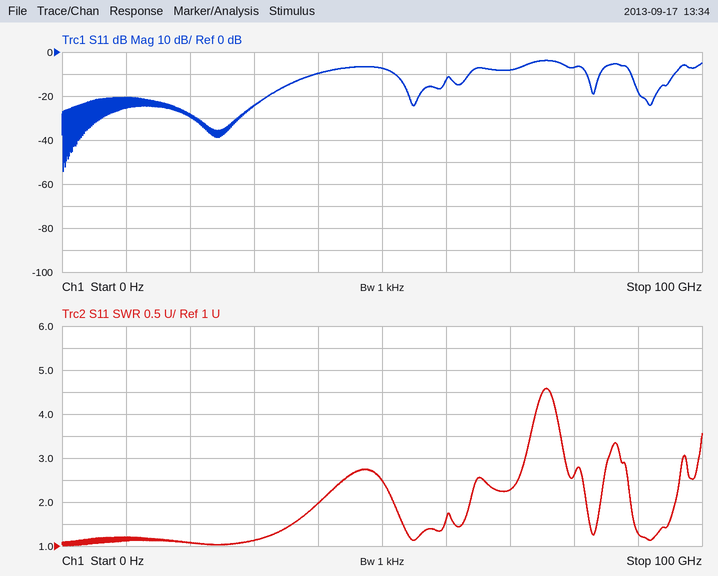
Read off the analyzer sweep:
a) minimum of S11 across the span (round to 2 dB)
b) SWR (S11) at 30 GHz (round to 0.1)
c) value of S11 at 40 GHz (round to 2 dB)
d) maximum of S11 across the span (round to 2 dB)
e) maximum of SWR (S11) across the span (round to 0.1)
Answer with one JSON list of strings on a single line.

["-54 dB", "1.1", "-10 dB", "-4 dB", "4.6"]
